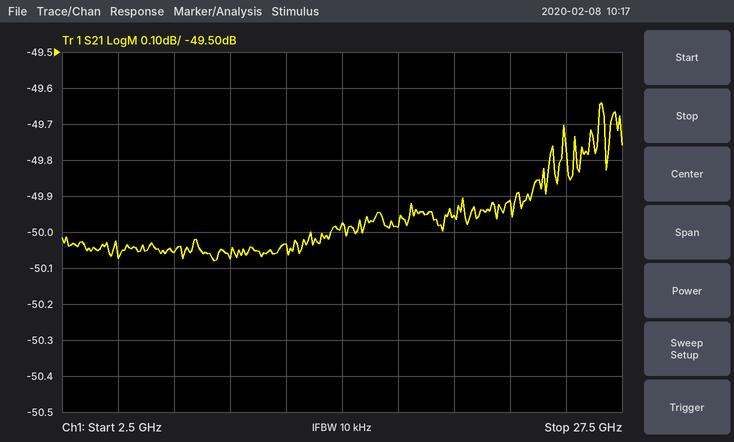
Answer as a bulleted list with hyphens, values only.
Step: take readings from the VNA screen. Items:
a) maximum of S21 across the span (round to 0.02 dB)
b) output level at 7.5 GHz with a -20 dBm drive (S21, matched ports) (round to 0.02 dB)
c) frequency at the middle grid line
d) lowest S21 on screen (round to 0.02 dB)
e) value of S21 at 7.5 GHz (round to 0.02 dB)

- -49.64 dB
- -70.06 dBm
- 15 GHz
- -50.08 dB
- -50.06 dB
